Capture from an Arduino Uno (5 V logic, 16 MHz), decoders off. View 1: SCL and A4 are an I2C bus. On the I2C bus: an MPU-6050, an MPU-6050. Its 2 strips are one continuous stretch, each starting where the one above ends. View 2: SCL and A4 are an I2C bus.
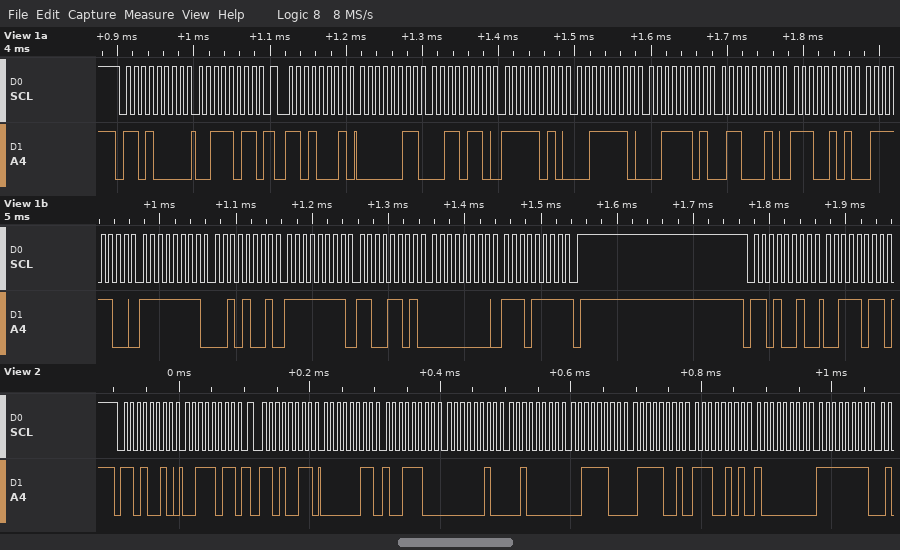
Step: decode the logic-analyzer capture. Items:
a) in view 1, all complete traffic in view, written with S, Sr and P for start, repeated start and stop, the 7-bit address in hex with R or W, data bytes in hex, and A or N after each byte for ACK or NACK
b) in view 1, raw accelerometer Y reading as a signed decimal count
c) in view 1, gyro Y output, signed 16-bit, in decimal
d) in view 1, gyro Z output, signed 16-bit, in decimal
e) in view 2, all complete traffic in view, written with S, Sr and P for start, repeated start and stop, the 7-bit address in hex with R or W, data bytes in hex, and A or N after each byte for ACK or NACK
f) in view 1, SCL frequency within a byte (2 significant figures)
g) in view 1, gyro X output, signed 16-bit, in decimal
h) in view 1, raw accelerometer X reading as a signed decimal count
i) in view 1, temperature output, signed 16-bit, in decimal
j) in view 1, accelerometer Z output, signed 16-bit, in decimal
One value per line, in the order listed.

S 68W A 3B A Sr 68R A 03 A 36 A FA A 3E A 3D A 62 A E5 A 7C A FF A 29 A FF A CD A 00 A EF N P S 69W A 3B A
-1474
-51
239
S 69W A 3B A Sr 69R A 03 A 9C A 02 A 20 A 3C A 79 A E5 A 80 A FF A
100 kHz
-215
822
-6788
15714
